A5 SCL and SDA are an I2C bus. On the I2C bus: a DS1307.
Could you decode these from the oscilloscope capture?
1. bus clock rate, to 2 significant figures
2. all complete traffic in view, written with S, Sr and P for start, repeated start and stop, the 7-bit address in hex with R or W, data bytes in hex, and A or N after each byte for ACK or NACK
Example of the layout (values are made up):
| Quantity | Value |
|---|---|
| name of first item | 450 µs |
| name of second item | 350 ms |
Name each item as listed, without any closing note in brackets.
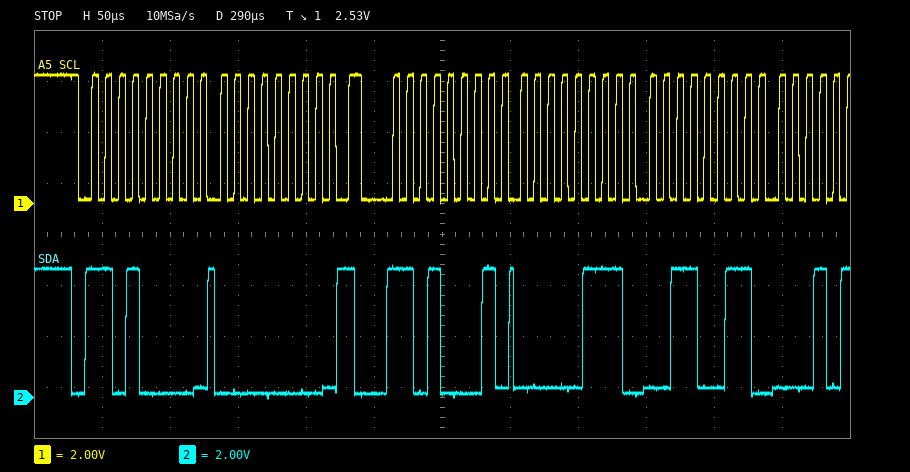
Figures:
| Quantity | Value |
|---|---|
| bus clock rate, to 2 significant figures | 100 kHz |
| all complete traffic in view, written with S, Sr and P for start, repeated start and stop, the 7-bit address in hex with R or W, data bytes in hex, and A or N after each byte for ACK or NACK | S 68W A 00 A Sr 68R A 07 A 33 A |
